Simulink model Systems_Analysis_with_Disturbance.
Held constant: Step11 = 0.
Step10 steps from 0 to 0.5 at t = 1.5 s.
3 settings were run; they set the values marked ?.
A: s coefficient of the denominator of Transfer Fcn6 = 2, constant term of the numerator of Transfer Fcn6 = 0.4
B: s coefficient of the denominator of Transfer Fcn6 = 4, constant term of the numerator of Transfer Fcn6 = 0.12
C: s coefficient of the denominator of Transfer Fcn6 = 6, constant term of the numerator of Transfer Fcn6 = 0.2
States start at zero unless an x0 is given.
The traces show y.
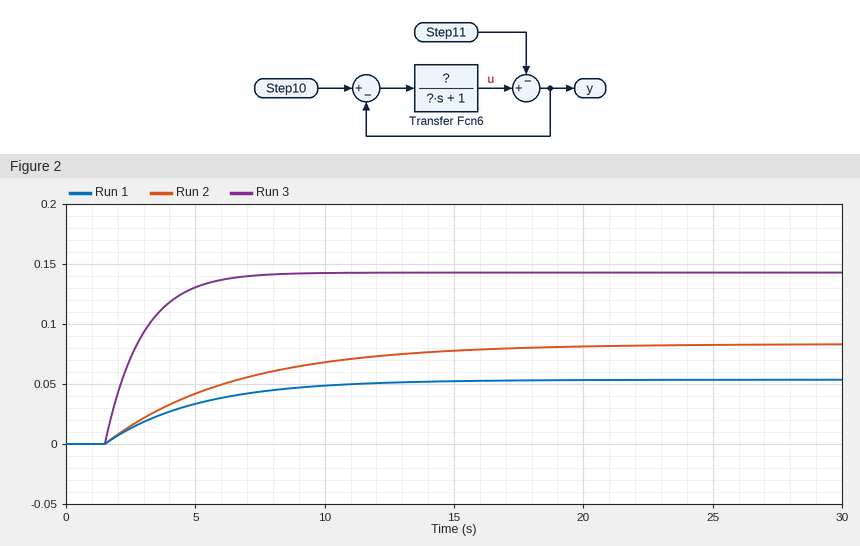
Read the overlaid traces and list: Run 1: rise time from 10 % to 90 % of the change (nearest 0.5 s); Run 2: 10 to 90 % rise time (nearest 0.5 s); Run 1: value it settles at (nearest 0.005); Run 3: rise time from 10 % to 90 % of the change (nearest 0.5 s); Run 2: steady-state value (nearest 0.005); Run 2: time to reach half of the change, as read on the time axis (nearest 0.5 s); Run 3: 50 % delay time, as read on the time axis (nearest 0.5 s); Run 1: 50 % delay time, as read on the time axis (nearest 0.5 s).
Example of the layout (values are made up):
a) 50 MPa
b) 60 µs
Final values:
a) 8.0 s
b) 11.0 s
c) 0.055
d) 3.0 s
e) 0.085
f) 5.0 s
g) 2.5 s
h) 4.0 s
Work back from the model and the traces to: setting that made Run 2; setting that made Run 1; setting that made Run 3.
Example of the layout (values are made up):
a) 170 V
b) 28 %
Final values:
a) C
b) B
c) A
